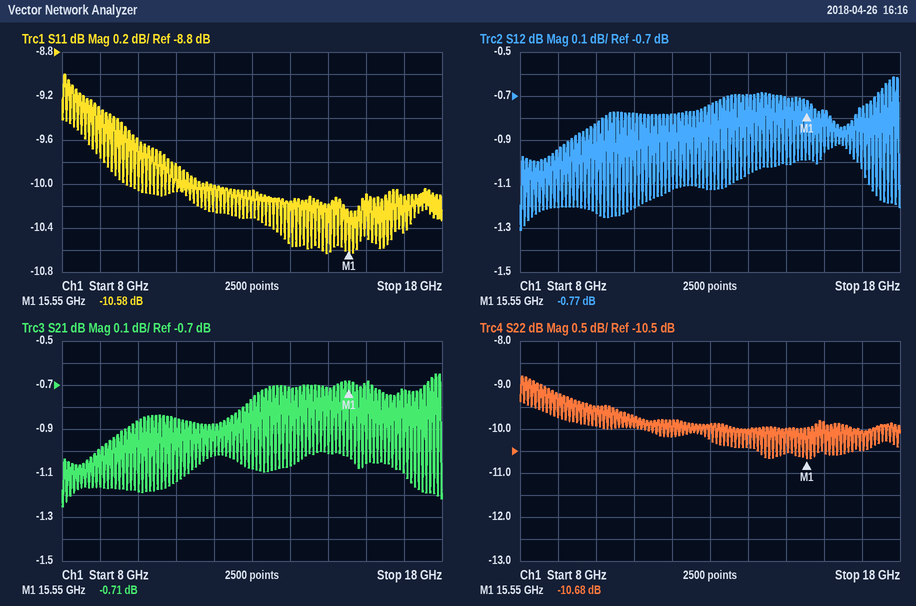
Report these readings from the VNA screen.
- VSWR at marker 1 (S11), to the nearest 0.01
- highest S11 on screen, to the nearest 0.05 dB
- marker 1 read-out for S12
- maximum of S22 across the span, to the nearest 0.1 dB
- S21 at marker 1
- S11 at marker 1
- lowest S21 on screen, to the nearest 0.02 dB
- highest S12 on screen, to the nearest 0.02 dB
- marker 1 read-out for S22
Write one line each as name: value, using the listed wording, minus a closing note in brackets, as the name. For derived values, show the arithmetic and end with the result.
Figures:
VSWR at marker 1 (S11), to the nearest 0.01: (1 + 0.2958)/(1 − 0.2958) ≈ 1.84
highest S11 on screen, to the nearest 0.05 dB: -9.00 dB
marker 1 read-out for S12: -0.77 dB
maximum of S22 across the span, to the nearest 0.1 dB: -8.8 dB
S21 at marker 1: -0.71 dB
S11 at marker 1: -10.58 dB
lowest S21 on screen, to the nearest 0.02 dB: -1.26 dB
highest S12 on screen, to the nearest 0.02 dB: -0.62 dB
marker 1 read-out for S22: -10.68 dB
